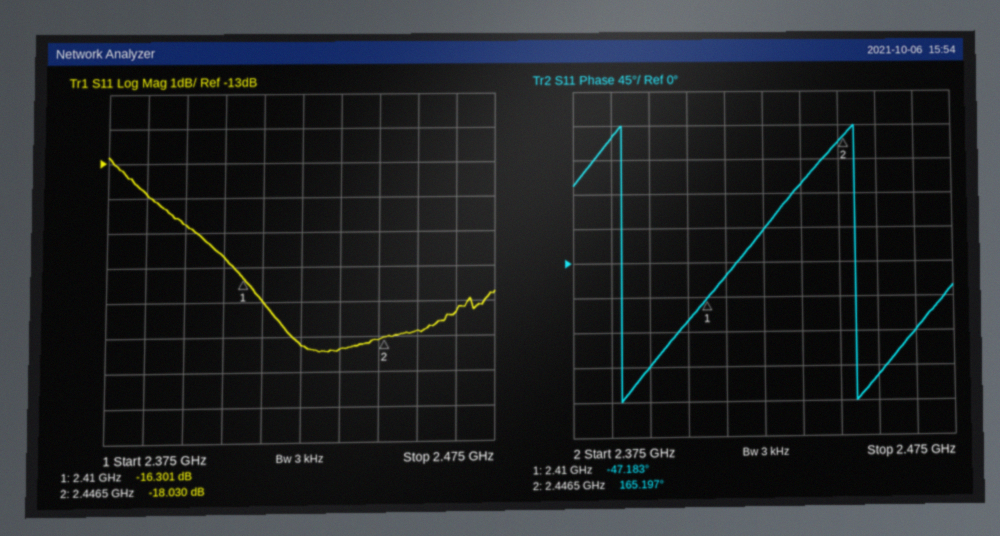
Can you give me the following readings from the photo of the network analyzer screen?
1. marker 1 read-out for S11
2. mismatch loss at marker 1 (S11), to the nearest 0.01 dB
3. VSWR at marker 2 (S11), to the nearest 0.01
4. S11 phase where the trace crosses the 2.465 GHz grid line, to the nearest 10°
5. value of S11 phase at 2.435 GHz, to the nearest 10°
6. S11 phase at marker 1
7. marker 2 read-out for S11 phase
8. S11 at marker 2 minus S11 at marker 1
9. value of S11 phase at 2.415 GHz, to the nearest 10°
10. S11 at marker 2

-16.301 dB
0.10 dB
1.29
-90°
100°
-47.183°
165.197°
-1.729 dB
-20°
-18.030 dB
